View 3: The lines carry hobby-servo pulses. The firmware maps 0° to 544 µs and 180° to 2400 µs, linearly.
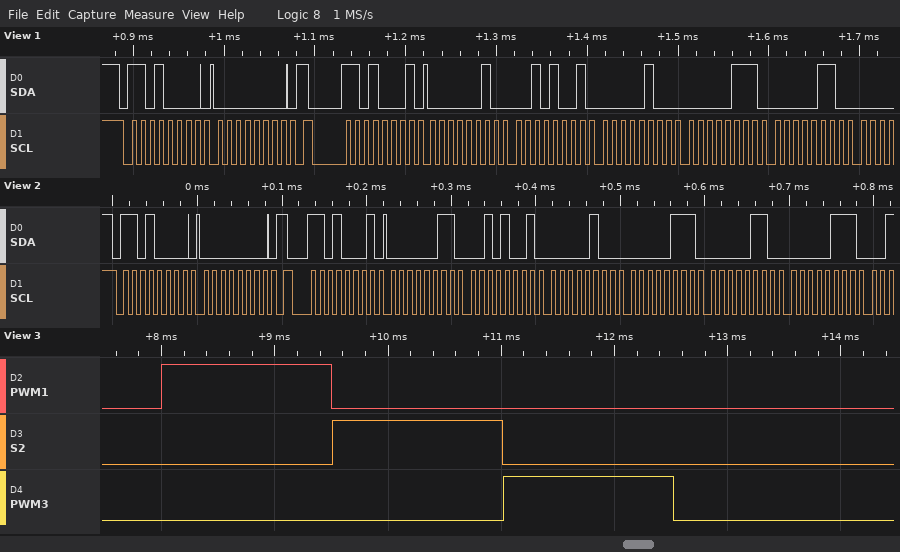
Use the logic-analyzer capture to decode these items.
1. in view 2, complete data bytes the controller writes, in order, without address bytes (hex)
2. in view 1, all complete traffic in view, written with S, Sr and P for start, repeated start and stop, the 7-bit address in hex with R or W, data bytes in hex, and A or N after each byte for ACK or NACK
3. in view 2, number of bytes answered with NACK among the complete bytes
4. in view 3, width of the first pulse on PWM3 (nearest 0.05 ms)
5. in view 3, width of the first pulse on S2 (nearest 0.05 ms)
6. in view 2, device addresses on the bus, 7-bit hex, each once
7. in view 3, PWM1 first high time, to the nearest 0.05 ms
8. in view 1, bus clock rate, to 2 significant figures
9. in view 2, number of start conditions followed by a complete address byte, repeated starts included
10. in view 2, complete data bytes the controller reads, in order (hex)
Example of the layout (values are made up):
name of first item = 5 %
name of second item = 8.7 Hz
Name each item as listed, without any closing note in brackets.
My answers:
in view 2, complete data bytes the controller writes, in order, without address bytes = 00
in view 1, all complete traffic in view, written with S, Sr and P for start, repeated start and stop, the 7-bit address in hex with R or W, data bytes in hex, and A or N after each byte for ACK or NACK = S 68W A 00 A Sr 68R A 02 A 29 A 04 A 07 A 06 A
in view 2, number of bytes answered with NACK among the complete bytes = 0
in view 3, width of the first pulse on PWM3 = 1.50 ms
in view 3, width of the first pulse on S2 = 1.50 ms
in view 2, device addresses on the bus, 7-bit hex, each once = 0x68
in view 3, PWM1 first high time, to the nearest 0.05 ms = 1.50 ms
in view 1, bus clock rate, to 2 significant figures = 100 kHz
in view 2, number of start conditions followed by a complete address byte, repeated starts included = 2
in view 2, complete data bytes the controller reads, in order = 03 29 04 07 06 07
